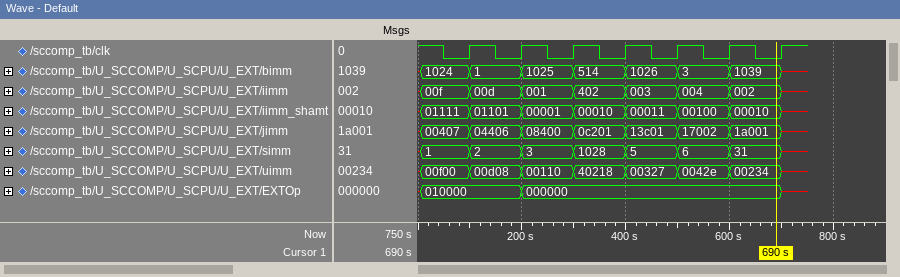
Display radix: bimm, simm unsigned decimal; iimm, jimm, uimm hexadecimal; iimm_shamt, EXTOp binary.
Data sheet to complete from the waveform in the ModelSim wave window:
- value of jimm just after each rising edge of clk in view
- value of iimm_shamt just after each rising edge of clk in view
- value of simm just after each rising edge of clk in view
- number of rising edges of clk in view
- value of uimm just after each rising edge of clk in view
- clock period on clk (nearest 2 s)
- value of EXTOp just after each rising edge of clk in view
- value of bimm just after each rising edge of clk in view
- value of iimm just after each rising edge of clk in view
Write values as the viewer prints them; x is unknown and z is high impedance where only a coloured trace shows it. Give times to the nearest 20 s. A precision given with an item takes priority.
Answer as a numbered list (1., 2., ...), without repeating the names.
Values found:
1. 04406, 08400, 0c201, 13c01, 17002, 1a001, x
2. 01101, 00001, 00010, 00011, 00100, 00010, x
3. 2, 3, 1028, 5, 6, 31, x
4. 7
5. 00d08, 00110, 40218, 00327, 0042e, 00234, x
6. 100 s
7. 010000, 000000, 000000, 000000, 000000, 000000, x
8. 1, 1025, 514, 1026, 3, 1039, x
9. 00d, 001, 402, 003, 004, 002, x
